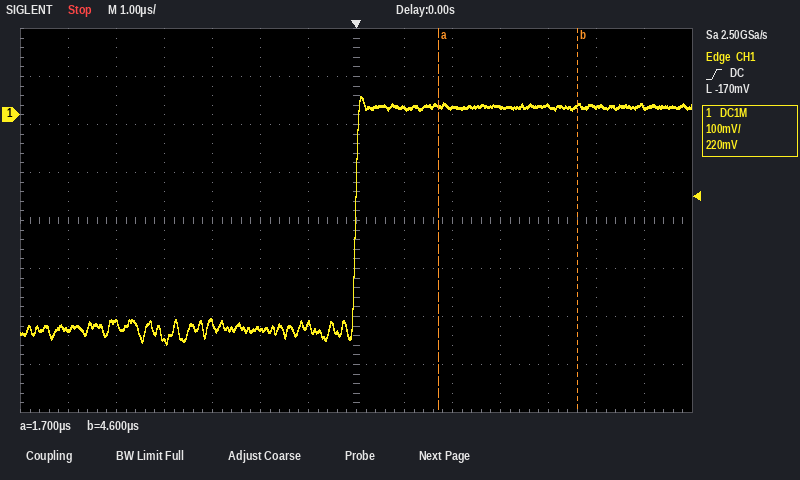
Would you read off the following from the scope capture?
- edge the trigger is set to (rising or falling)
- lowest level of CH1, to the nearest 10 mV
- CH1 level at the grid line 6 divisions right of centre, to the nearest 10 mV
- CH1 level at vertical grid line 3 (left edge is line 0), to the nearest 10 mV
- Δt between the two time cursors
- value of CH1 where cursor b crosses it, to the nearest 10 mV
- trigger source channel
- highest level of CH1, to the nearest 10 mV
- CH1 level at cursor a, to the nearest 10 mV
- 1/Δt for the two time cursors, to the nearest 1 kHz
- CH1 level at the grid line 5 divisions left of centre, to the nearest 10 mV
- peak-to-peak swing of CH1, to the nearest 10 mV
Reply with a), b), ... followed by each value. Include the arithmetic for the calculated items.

a) rising
b) -480 mV
c) 20 mV
d) -470 mV
e) 4.6 µs − (1.7 µs) = 2.9 µs
f) 20 mV
g) CH1
h) 40 mV
i) 20 mV
j) 1 / 2.9 µs ≈ 345 kHz
k) -430 mV
l) 40 mV − (-480 mV) = 520 mV
